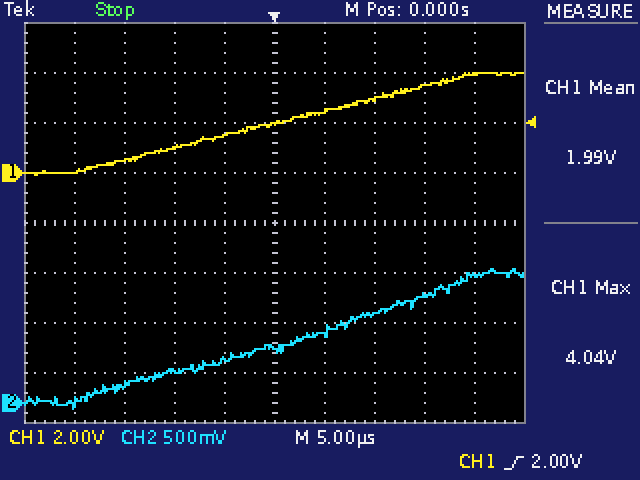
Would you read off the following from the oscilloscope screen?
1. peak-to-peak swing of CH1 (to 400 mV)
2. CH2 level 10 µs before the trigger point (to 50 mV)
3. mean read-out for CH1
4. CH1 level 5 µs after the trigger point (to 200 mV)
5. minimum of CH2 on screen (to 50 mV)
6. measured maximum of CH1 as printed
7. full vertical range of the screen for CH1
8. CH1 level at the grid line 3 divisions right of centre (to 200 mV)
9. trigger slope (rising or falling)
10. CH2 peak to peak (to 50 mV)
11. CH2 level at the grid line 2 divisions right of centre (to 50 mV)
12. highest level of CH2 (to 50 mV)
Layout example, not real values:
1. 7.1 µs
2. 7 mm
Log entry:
1. 4.0 V
2. 300 mV
3. 1.99 V
4. 2.4 V
5. -50 mV
6. 4.04 V
7. 16 V
8. 3.4 V
9. rising
10. 1.40 V
11. 900 mV
12. 1.35 V
